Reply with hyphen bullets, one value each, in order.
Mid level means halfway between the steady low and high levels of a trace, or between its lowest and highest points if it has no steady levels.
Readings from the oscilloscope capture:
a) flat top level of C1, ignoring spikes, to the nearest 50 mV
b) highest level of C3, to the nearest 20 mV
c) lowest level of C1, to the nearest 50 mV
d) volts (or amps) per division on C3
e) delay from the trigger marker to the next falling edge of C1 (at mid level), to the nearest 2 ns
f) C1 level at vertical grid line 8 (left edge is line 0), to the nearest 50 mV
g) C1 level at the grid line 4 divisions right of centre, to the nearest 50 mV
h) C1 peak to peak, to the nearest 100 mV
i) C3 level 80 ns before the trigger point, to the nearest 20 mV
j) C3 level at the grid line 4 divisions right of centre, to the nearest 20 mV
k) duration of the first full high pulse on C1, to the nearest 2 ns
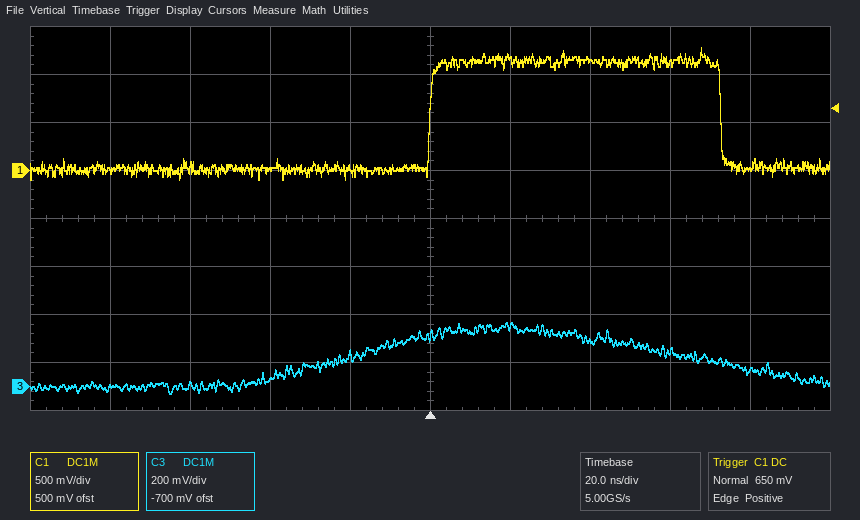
- 1.15 V
- 260 mV
- -100 mV
- 200 mV
- 72 ns
- 1.15 V
- 50 mV
- 1.40 V
- 0 mV
- 60 mV
- 72 ns
